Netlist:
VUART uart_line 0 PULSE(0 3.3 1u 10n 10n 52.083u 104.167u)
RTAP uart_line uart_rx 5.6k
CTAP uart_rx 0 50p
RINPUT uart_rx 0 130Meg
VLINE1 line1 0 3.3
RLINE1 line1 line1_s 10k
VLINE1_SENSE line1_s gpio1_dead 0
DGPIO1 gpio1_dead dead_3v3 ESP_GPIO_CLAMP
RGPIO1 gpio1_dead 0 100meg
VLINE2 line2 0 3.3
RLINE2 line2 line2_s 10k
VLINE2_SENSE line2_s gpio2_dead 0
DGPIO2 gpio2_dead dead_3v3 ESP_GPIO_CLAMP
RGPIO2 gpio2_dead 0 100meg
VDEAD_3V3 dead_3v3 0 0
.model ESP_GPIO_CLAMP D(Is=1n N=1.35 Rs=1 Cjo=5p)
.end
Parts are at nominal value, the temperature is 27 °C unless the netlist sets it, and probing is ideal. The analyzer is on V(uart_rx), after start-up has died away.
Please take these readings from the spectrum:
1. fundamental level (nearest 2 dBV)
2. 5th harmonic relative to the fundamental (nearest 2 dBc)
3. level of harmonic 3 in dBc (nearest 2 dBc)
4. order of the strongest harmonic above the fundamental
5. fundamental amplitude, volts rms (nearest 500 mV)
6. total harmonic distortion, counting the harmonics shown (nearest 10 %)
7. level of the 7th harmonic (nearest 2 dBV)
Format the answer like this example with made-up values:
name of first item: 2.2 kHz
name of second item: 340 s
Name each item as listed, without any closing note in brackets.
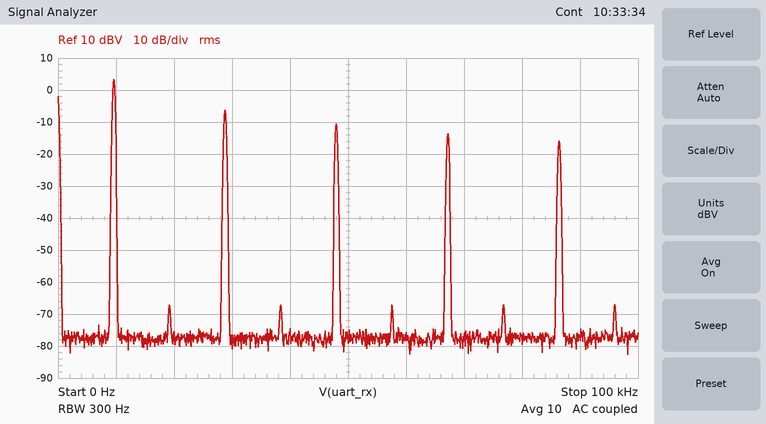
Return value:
fundamental level: 4 dBV
5th harmonic relative to the fundamental: -14 dBc
level of harmonic 3 in dBc: -10 dBc
order of the strongest harmonic above the fundamental: 3
fundamental amplitude, volts rms: 1.5 V
total harmonic distortion, counting the harmonics shown: 40 %
level of the 7th harmonic: -14 dBV
